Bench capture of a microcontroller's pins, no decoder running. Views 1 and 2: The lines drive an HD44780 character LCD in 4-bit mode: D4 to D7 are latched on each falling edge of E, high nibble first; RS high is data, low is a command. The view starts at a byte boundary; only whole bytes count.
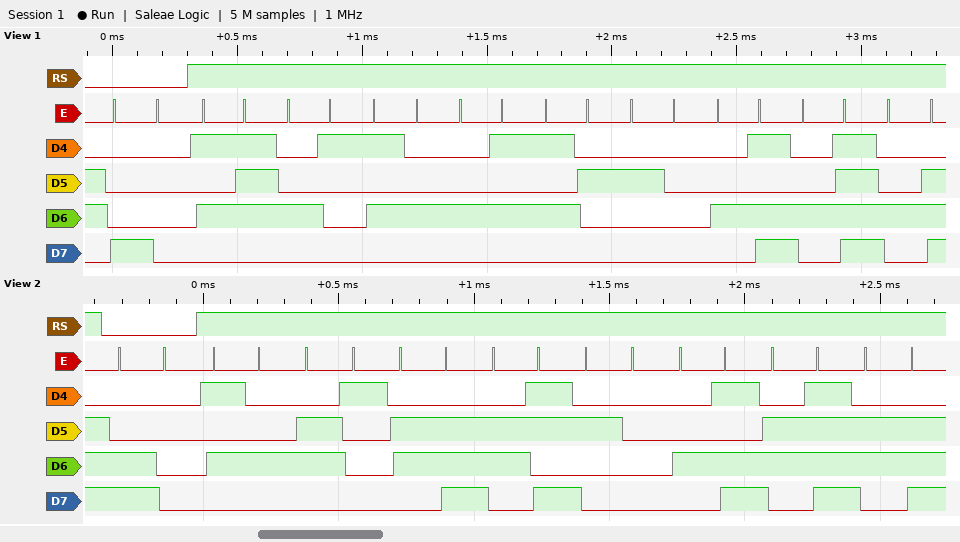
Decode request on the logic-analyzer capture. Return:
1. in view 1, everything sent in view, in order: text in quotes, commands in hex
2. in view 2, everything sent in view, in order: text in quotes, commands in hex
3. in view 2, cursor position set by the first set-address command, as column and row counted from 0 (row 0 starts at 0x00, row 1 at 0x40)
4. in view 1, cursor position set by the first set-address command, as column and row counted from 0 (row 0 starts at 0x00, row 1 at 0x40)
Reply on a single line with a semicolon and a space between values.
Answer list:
0x80 "WATER MON"; 0xC0 "Tank Mon"; column 0, row 1; column 0, row 0
